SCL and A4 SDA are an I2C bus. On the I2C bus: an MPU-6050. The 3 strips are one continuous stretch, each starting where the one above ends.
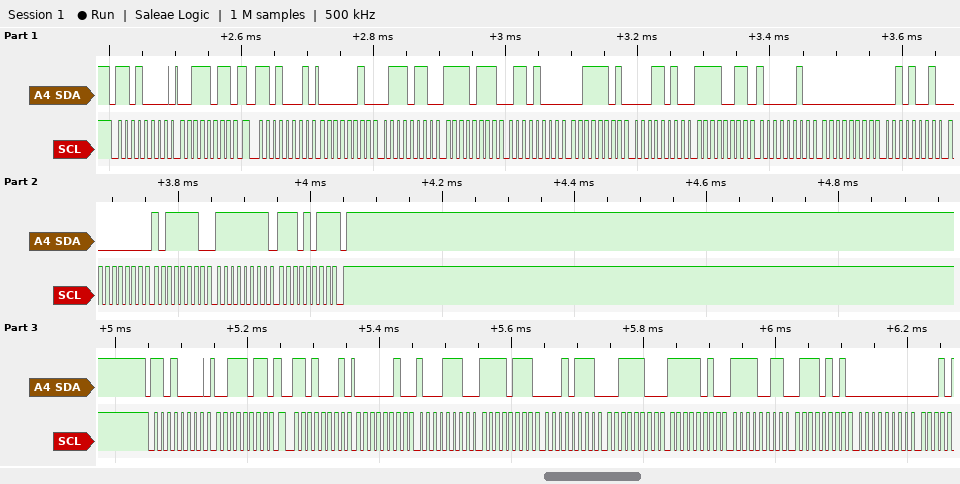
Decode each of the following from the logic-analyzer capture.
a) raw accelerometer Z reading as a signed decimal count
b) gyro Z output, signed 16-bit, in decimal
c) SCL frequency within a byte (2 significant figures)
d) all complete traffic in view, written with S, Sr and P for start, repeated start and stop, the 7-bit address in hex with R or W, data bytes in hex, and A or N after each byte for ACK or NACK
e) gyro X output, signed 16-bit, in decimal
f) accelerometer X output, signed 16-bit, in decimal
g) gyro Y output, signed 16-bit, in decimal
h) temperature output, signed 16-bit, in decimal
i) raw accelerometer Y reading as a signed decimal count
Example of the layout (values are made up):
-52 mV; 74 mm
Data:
15642; -21; 100 kHz; S 68W A 3B A Sr 68R A 02 A 76 A F7 A 68 A 3D A 1A A F3 A 82 A 00 A 29 A 00 A BE A FF A EB N P S 68W A 3B A Sr 68R A 02 A 8E A F7 A 17 A 3C A FA A F3 A 75 A 00 A; 41; 630; 190; -3198; -2200
